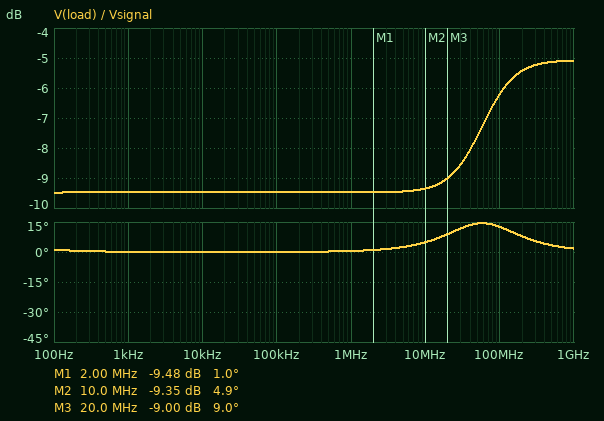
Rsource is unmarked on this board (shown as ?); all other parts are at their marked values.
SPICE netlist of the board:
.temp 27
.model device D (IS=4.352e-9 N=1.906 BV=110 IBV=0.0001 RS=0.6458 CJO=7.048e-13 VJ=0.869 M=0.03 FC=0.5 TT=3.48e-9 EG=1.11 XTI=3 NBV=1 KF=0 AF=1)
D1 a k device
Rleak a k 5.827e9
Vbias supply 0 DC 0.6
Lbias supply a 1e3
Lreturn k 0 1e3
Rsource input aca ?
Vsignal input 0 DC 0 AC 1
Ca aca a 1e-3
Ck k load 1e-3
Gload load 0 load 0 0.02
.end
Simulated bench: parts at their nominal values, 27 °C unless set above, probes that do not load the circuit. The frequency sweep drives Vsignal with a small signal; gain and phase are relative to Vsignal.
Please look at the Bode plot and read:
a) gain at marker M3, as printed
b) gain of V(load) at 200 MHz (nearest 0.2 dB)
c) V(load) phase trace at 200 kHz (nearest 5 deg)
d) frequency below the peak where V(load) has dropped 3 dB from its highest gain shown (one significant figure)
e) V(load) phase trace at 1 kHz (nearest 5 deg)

-9.00 dB
-5.4 dB
0 deg
40 MHz
0 deg
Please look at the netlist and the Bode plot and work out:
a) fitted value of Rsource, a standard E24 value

39 Ω
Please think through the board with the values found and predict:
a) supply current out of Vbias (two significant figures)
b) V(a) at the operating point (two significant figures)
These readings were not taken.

830 µA
600 mV
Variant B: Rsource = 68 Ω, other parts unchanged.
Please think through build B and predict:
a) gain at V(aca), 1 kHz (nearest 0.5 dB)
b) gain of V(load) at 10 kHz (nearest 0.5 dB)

-4.0 dB
-11.0 dB
